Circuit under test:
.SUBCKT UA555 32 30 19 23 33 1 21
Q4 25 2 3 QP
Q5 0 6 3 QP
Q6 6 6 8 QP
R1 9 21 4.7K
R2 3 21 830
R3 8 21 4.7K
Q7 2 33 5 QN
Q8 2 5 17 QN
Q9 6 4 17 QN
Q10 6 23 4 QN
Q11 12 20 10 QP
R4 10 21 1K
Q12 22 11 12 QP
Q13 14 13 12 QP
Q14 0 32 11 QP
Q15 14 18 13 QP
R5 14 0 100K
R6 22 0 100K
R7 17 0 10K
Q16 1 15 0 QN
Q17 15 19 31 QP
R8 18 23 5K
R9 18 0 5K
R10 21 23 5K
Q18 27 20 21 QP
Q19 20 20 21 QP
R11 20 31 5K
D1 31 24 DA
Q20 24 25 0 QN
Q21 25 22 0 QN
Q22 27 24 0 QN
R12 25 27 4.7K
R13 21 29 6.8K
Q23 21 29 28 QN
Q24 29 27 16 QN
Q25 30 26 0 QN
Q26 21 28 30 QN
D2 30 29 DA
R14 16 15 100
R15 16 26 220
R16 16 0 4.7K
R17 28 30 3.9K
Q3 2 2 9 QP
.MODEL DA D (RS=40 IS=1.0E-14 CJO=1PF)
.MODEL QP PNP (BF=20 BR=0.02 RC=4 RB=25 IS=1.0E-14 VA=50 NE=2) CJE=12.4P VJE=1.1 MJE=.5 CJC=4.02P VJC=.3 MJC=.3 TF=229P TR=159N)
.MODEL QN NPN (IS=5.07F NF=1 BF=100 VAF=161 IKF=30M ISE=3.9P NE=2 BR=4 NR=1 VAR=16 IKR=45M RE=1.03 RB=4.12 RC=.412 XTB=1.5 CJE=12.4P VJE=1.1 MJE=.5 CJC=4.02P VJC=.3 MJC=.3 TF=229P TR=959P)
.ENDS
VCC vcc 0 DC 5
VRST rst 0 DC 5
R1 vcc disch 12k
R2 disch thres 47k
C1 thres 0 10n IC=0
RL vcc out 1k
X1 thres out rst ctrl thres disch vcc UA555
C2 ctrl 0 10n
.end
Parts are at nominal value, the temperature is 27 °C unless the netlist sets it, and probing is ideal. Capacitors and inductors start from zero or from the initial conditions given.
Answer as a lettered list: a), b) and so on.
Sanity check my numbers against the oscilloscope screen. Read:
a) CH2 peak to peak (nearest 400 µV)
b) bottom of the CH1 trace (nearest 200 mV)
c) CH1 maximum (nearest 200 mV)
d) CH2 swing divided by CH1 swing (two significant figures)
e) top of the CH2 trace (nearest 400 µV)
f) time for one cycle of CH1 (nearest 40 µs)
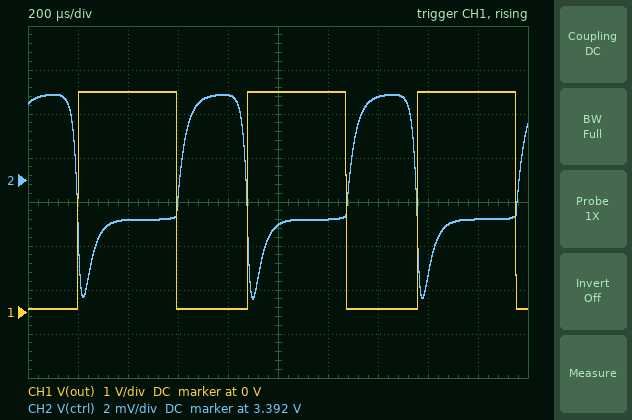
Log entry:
a) 9.2 mV
b) 0 V
c) 5.0 V
d) 0.0019
e) 3.3960 V
f) 680 µs
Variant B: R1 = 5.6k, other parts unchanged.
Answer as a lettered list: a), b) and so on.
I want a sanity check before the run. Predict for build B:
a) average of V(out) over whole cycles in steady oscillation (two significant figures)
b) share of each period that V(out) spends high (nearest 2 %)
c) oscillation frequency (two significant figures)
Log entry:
a) 2.8 V
b) 56 %
c) 1.6 kHz
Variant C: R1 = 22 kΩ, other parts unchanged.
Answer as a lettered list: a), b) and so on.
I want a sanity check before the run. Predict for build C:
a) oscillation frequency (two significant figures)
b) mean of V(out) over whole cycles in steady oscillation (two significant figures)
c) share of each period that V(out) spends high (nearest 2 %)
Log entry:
a) 1.3 kHz
b) 3.1 V
c) 62 %
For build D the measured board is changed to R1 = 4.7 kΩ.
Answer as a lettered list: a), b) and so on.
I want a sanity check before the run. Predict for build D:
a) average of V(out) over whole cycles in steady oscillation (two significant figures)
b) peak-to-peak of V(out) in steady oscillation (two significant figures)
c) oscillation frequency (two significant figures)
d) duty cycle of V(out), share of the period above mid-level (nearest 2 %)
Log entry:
a) 2.8 V
b) 5.0 V
c) 1.6 kHz
d) 54 %
